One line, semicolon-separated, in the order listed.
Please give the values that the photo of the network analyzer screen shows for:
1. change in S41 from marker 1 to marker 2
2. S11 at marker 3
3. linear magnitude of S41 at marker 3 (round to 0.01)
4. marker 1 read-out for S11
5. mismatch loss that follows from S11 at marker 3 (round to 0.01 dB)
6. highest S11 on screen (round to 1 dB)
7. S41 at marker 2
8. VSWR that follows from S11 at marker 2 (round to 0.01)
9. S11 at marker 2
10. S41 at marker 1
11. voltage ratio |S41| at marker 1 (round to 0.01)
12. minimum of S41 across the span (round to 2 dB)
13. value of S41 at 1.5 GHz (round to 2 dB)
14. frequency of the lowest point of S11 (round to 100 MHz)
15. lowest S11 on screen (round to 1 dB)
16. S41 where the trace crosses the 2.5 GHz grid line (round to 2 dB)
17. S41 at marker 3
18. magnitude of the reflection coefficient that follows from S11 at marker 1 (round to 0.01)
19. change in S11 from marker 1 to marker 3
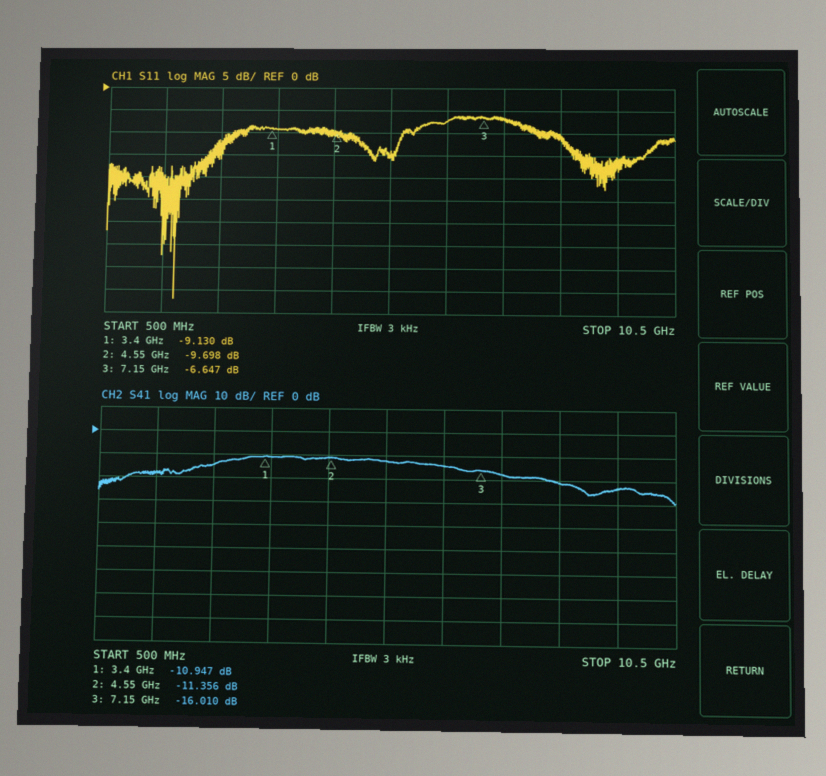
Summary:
-0.409 dB; -6.647 dB; 0.16; -9.130 dB; 1.06 dB; -6 dB; -11.356 dB; 1.97; -9.698 dB; -10.947 dB; 0.28; -30 dB; -18 dB; 1.7 GHz; -47 dB; -14 dB; -16.010 dB; 0.35; 2.483 dB
